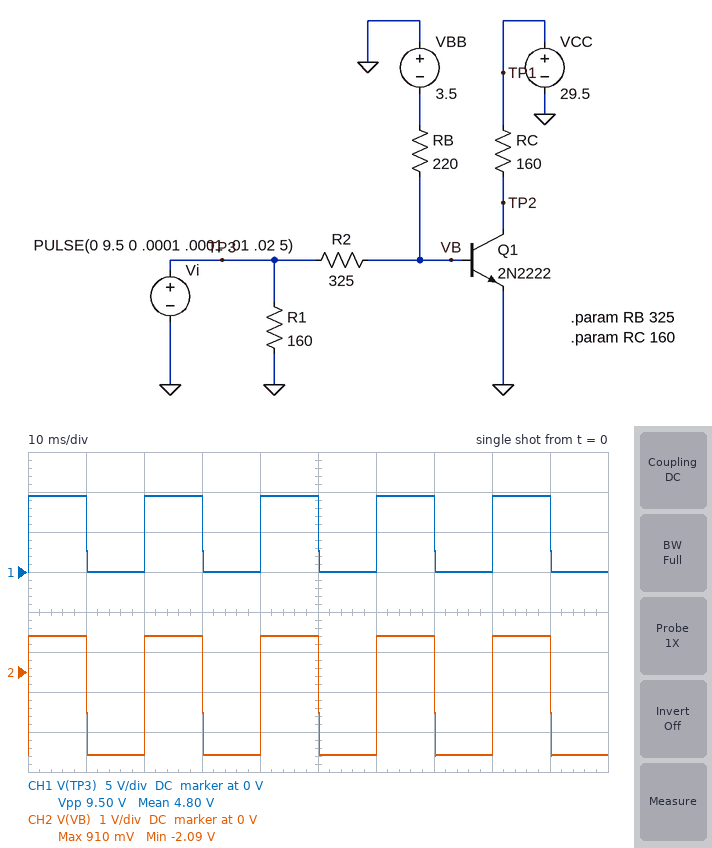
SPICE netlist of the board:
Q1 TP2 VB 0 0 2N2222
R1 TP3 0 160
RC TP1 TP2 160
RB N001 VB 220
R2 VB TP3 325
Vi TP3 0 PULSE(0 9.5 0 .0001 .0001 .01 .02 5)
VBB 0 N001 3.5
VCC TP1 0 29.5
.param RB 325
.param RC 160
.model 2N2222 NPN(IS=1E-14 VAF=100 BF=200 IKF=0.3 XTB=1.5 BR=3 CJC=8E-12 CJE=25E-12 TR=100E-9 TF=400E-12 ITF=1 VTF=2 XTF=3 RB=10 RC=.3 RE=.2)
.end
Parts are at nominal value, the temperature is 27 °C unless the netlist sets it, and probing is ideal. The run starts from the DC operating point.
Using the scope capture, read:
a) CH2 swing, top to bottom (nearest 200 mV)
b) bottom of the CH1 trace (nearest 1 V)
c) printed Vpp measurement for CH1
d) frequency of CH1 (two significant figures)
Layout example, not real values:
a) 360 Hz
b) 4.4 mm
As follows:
a) 3.0 V
b) 0 V
c) 9.50 V
d) 50 Hz
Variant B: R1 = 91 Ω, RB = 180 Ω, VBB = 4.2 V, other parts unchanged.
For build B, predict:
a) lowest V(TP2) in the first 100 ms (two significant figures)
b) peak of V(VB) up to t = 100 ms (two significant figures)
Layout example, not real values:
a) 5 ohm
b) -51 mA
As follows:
a) 29 V
b) 680 mV
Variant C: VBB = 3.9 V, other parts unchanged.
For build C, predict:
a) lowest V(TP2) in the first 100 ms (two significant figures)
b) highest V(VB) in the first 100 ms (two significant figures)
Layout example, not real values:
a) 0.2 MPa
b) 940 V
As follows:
a) 180 mV
b) 890 mV
